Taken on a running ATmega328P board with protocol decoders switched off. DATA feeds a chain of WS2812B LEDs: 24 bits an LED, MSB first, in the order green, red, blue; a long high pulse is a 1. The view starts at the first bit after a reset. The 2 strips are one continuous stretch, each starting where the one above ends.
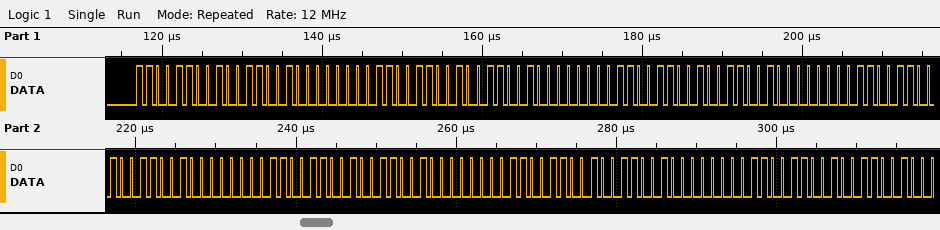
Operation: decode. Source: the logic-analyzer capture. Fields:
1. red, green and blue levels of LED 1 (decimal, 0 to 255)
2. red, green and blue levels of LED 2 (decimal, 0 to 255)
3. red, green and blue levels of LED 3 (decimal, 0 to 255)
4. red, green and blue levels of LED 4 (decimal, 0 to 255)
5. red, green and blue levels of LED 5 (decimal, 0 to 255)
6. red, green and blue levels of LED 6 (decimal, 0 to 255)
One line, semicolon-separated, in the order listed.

153, 204, 0; 153, 204, 0; 153, 204, 0; 153, 204, 0; 153, 204, 0; 153, 204, 0
